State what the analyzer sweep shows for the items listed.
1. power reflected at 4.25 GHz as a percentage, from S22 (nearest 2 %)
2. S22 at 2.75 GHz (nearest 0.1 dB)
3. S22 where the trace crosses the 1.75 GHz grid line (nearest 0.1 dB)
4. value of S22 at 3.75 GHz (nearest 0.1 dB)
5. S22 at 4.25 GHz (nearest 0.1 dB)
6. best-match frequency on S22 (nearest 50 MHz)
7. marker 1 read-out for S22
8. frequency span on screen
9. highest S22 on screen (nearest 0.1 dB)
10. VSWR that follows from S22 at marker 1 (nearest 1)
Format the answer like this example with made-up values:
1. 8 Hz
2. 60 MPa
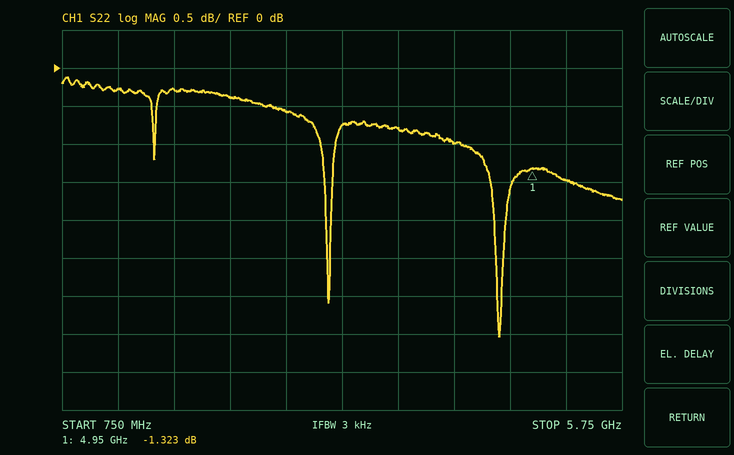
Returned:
1. 80 %
2. -0.6 dB
3. -0.3 dB
4. -0.8 dB
5. -1.0 dB
6. 4.65 GHz
7. -1.323 dB
8. 5 GHz
9. -0.1 dB
10. 13
